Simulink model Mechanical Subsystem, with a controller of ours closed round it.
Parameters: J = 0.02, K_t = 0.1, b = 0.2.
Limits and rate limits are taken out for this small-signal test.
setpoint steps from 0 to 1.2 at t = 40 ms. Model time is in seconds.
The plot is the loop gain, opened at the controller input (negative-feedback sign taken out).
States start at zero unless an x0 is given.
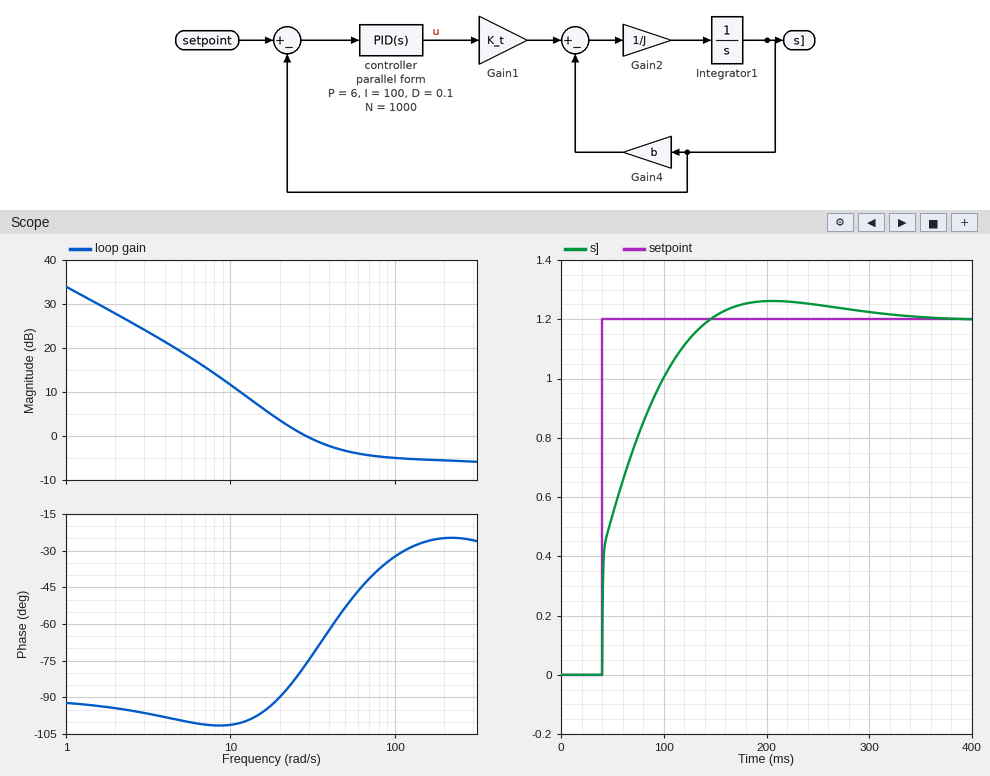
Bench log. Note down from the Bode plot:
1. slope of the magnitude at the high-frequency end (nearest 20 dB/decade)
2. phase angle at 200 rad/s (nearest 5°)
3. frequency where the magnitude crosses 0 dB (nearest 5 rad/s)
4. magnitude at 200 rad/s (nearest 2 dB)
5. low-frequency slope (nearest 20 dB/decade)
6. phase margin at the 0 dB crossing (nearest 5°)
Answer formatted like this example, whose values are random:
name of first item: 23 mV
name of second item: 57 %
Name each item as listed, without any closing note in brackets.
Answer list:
slope of the magnitude at the high-frequency end: 0 dB/decade
phase angle at 200 rad/s: -25°
frequency where the magnitude crosses 0 dB: 30 rad/s
magnitude at 200 rad/s: -6 dB
low-frequency slope: -20 dB/decade
phase margin at the 0 dB crossing: 105°
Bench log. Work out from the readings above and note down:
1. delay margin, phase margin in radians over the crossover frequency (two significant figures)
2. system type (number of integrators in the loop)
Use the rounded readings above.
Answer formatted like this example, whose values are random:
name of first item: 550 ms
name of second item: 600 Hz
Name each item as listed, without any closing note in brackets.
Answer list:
delay margin, phase margin in radians over the crossover frequency: 0.061 s
system type: 1
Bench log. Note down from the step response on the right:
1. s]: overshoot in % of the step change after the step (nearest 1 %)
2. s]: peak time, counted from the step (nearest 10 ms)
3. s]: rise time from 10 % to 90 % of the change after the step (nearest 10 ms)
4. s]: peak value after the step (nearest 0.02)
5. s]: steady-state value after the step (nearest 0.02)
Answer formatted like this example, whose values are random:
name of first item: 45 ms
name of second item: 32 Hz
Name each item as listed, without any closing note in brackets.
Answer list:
s]: overshoot in % of the step change after the step: 5 %
s]: peak time, counted from the step: 170 ms
s]: rise time from 10 % to 90 % of the change after the step: 70 ms
s]: peak value after the step: 1.26
s]: steady-state value after the step: 1.20
